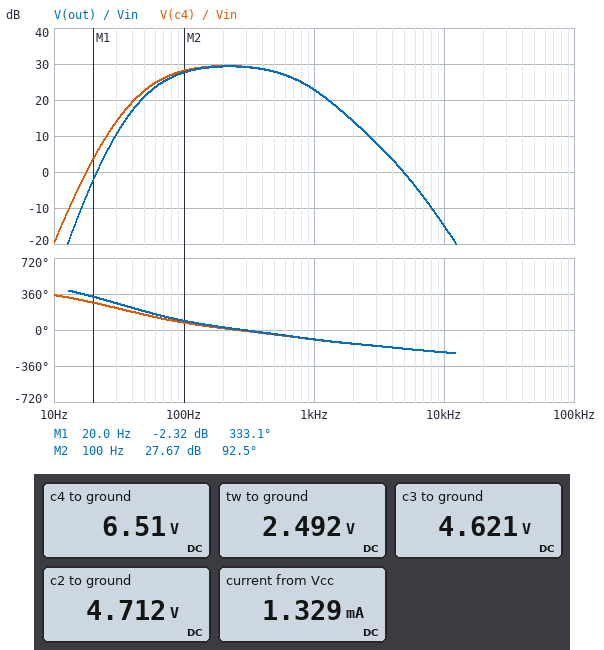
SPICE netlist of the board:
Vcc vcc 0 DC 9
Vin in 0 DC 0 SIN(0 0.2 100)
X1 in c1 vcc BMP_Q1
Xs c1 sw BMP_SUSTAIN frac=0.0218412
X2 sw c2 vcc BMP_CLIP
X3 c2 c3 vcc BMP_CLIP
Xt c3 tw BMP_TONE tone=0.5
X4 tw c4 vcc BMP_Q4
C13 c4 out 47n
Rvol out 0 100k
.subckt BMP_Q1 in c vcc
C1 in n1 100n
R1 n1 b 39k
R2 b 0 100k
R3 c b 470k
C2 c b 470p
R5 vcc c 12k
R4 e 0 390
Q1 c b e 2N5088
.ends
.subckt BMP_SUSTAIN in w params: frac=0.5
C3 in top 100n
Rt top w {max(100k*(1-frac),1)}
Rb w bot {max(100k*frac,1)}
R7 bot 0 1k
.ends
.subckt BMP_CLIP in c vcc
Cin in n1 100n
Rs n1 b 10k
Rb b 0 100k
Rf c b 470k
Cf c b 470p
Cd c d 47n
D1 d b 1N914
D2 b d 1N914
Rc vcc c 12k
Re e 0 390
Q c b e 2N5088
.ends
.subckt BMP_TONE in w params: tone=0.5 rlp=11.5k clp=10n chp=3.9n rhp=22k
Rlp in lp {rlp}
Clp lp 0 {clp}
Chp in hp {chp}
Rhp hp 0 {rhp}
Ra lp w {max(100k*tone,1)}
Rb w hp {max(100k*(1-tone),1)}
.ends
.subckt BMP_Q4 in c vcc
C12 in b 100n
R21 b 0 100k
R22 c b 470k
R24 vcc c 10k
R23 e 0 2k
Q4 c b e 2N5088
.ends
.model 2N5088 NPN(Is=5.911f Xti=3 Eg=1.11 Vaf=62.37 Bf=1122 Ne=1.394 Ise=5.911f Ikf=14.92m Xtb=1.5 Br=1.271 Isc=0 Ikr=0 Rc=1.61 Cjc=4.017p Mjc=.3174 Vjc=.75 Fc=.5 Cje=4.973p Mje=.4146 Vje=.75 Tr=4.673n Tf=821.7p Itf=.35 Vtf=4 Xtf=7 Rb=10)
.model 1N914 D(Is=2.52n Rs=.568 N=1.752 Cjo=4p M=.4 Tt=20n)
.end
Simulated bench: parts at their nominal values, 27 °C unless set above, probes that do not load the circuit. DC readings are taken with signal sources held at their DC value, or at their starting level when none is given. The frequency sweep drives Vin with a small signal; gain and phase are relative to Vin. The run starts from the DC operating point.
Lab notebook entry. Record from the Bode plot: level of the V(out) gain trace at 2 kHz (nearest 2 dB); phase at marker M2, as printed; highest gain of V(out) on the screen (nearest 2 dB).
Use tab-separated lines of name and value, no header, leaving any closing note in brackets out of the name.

level of the V(out) gain trace at 2 kHz	14 dB
phase at marker M2, as printed	92.5 deg
highest gain of V(out) on the screen	30 dB
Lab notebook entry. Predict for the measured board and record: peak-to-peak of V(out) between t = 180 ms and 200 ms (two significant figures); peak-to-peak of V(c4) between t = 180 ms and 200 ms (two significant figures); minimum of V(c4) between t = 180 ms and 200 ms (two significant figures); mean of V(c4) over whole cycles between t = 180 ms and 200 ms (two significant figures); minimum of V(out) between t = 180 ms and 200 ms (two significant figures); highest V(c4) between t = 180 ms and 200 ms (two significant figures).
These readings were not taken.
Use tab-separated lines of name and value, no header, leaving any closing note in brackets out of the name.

peak-to-peak of V(out) between t = 180 ms and 200 ms	1.4 V
peak-to-peak of V(c4) between t = 180 ms and 200 ms	1.5 V
minimum of V(c4) between t = 180 ms and 200 ms	5.7 V
mean of V(c4) over whole cycles between t = 180 ms and 200 ms	6.5 V
minimum of V(out) between t = 180 ms and 200 ms	-690 mV
highest V(c4) between t = 180 ms and 200 ms	7.3 V
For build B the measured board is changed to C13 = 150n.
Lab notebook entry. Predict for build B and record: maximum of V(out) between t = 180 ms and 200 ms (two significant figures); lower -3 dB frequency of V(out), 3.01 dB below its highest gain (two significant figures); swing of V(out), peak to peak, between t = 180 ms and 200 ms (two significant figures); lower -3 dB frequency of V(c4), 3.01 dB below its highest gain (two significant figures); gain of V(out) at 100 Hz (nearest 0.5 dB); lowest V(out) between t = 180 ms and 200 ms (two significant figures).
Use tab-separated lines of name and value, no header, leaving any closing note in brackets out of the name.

maximum of V(out) between t = 180 ms and 200 ms	730 mV
lower -3 dB frequency of V(out), 3.01 dB below its highest gain	75 Hz
swing of V(out), peak to peak, between t = 180 ms and 200 ms	1.5 V
lower -3 dB frequency of V(c4), 3.01 dB below its highest gain	74 Hz
gain of V(out) at 100 Hz	28.0 dB
lowest V(out) between t = 180 ms and 200 ms	-740 mV
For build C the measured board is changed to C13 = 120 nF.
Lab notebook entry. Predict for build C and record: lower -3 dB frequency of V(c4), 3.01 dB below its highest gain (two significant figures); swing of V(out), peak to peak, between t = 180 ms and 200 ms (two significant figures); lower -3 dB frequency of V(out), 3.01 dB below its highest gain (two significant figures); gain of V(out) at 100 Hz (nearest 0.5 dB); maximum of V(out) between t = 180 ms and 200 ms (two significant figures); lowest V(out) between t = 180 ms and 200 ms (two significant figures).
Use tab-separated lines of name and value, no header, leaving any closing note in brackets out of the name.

lower -3 dB frequency of V(c4), 3.01 dB below its highest gain	74 Hz
swing of V(out), peak to peak, between t = 180 ms and 200 ms	1.5 V
lower -3 dB frequency of V(out), 3.01 dB below its highest gain	75 Hz
gain of V(out) at 100 Hz	28.0 dB
maximum of V(out) between t = 180 ms and 200 ms	730 mV
lowest V(out) between t = 180 ms and 200 ms	-730 mV
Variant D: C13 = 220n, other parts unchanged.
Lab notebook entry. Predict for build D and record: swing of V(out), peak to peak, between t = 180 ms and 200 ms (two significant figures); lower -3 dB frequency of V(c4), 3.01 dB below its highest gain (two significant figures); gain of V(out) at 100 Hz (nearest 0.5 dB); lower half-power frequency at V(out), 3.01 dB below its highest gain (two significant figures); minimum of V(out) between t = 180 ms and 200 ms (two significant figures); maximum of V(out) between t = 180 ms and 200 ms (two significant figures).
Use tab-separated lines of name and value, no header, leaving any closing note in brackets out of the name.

swing of V(out), peak to peak, between t = 180 ms and 200 ms	1.5 V
lower -3 dB frequency of V(c4), 3.01 dB below its highest gain	74 Hz
gain of V(out) at 100 Hz	28.0 dB
lower half-power frequency at V(out), 3.01 dB below its highest gain	75 Hz
minimum of V(out) between t = 180 ms and 200 ms	-740 mV
maximum of V(out) between t = 180 ms and 200 ms	740 mV
